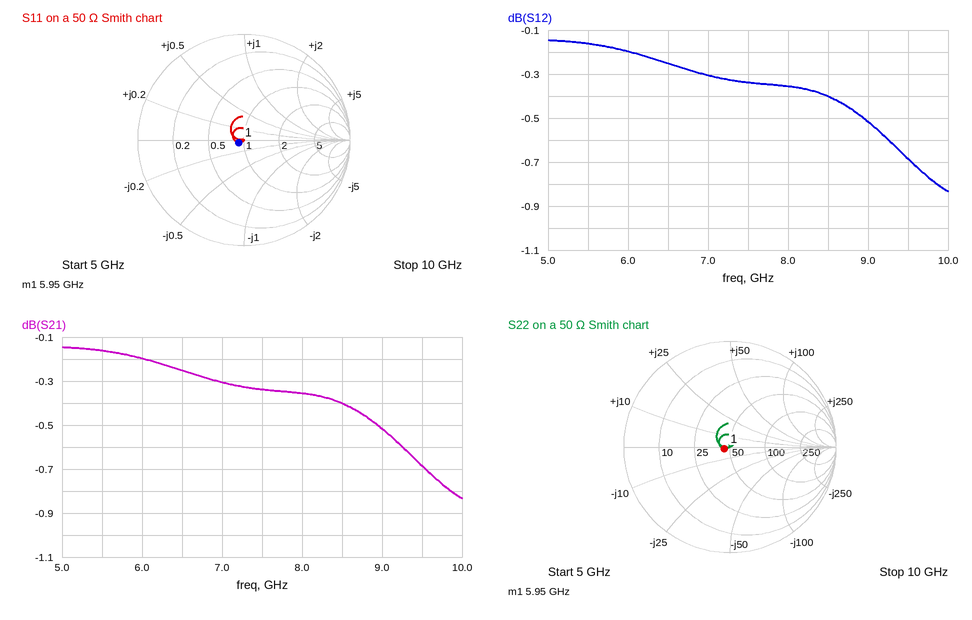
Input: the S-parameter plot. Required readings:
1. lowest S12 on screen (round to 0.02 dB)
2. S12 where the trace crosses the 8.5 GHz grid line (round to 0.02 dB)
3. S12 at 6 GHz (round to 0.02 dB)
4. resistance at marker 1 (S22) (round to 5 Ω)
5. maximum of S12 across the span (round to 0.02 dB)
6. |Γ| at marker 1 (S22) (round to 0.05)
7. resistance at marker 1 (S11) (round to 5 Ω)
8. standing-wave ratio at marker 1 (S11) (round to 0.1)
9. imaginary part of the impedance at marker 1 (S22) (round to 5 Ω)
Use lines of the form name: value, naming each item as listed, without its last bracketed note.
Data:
lowest S12 on screen: -0.84 dB
S12 where the trace crosses the 8.5 GHz grid line: -0.40 dB
S12 at 6 GHz: -0.20 dB
resistance at marker 1 (S22): 45 Ω
maximum of S12 across the span: -0.14 dB
|Γ| at marker 1 (S22): 0.05
resistance at marker 1 (S11): 45 Ω
standing-wave ratio at marker 1 (S11): 1.1
imaginary part of the impedance at marker 1 (S22): 0 Ω
